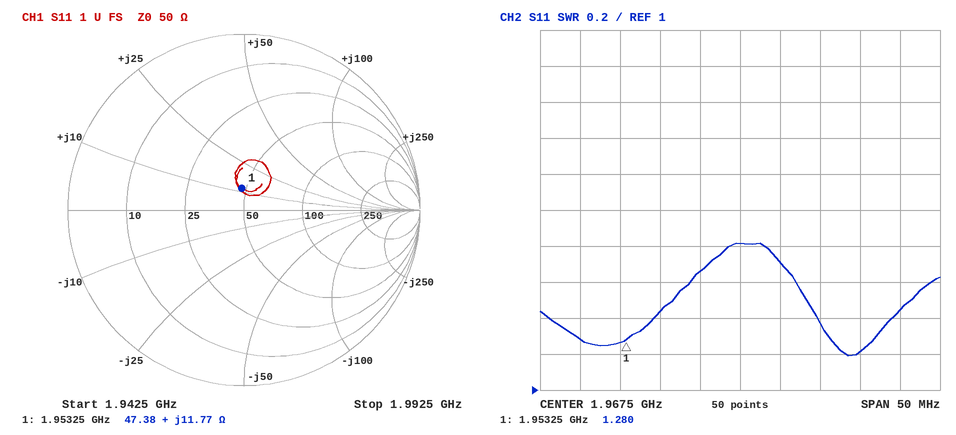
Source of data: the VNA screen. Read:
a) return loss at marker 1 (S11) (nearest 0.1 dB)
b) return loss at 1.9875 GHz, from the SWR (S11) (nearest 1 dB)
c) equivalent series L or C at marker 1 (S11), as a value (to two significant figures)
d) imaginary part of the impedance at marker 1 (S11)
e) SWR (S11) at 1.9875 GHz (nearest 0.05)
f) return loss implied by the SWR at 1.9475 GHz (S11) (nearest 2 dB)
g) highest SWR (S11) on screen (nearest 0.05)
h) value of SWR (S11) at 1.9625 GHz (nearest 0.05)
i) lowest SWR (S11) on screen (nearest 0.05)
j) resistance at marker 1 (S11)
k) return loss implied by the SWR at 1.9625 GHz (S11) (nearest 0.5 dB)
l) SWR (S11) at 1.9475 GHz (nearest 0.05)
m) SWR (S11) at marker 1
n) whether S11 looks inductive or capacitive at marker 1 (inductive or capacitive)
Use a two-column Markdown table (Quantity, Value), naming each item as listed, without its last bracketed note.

| Quantity | Value |
|---|---|
| return loss at marker 1 (S11) | 18.2 dB |
| return loss at 1.9875 GHz, from the SWR (S11) | 15 dB |
| equivalent series L or C at marker 1 (S11), as a value | 960 pH |
| imaginary part of the impedance at marker 1 | +11.77 Ω |
| SWR (S11) at 1.9875 GHz | 1.45 |
| return loss implied by the SWR at 1.9475 GHz (S11) | 18 dB |
| highest SWR (S11) on screen | 1.80 |
| value of SWR (S11) at 1.9625 GHz | 1.65 |
| lowest SWR (S11) on screen | 1.20 |
| resistance at marker 1 | 47.38 Ω |
| return loss implied by the SWR at 1.9625 GHz (S11) | 12.0 dB |
| SWR (S11) at 1.9475 GHz | 1.30 |
| SWR (S11) at marker 1 | 1.280 |
| whether S11 looks inductive or capacitive at marker 1 | inductive |
